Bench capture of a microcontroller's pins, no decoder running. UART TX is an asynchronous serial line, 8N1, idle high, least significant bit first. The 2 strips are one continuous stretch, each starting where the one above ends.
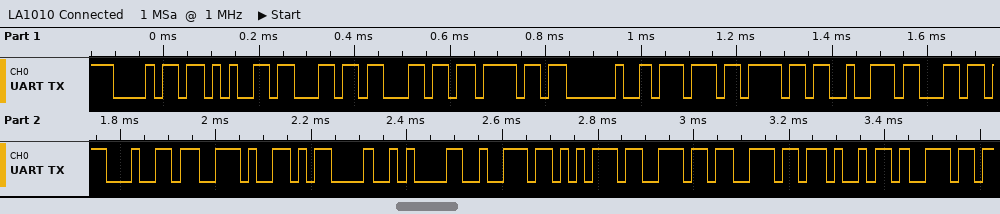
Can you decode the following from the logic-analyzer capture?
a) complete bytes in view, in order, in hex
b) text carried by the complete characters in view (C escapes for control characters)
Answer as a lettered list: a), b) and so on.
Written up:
a) 68 65 6C 6C 6F 20 77 6F 72 6C 64 2E 0D 0A 72 75 6E 6E 69 6E
b) "hello world.\r\nrunnin"
